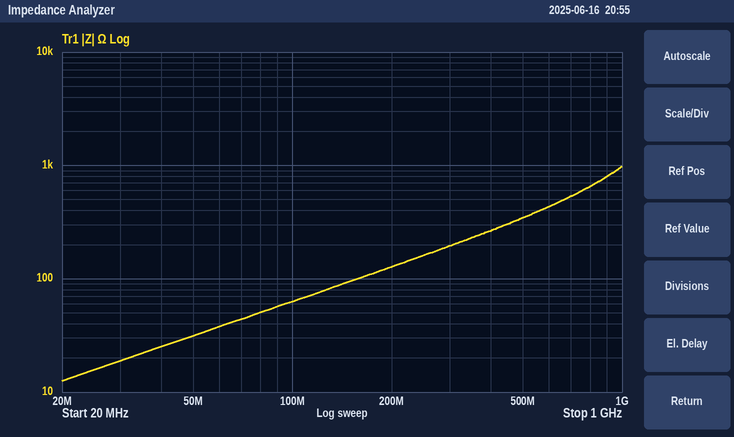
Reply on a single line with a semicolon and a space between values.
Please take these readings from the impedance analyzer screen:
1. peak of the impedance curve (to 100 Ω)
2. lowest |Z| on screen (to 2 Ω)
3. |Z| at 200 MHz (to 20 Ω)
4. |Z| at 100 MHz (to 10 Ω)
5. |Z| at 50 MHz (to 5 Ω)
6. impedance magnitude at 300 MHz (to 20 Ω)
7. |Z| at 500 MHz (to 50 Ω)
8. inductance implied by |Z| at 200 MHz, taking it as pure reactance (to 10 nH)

1.0 kΩ; 12 Ω; 120 Ω; 60 Ω; 30 Ω; 200 Ω; 350 Ω; 100 nH
